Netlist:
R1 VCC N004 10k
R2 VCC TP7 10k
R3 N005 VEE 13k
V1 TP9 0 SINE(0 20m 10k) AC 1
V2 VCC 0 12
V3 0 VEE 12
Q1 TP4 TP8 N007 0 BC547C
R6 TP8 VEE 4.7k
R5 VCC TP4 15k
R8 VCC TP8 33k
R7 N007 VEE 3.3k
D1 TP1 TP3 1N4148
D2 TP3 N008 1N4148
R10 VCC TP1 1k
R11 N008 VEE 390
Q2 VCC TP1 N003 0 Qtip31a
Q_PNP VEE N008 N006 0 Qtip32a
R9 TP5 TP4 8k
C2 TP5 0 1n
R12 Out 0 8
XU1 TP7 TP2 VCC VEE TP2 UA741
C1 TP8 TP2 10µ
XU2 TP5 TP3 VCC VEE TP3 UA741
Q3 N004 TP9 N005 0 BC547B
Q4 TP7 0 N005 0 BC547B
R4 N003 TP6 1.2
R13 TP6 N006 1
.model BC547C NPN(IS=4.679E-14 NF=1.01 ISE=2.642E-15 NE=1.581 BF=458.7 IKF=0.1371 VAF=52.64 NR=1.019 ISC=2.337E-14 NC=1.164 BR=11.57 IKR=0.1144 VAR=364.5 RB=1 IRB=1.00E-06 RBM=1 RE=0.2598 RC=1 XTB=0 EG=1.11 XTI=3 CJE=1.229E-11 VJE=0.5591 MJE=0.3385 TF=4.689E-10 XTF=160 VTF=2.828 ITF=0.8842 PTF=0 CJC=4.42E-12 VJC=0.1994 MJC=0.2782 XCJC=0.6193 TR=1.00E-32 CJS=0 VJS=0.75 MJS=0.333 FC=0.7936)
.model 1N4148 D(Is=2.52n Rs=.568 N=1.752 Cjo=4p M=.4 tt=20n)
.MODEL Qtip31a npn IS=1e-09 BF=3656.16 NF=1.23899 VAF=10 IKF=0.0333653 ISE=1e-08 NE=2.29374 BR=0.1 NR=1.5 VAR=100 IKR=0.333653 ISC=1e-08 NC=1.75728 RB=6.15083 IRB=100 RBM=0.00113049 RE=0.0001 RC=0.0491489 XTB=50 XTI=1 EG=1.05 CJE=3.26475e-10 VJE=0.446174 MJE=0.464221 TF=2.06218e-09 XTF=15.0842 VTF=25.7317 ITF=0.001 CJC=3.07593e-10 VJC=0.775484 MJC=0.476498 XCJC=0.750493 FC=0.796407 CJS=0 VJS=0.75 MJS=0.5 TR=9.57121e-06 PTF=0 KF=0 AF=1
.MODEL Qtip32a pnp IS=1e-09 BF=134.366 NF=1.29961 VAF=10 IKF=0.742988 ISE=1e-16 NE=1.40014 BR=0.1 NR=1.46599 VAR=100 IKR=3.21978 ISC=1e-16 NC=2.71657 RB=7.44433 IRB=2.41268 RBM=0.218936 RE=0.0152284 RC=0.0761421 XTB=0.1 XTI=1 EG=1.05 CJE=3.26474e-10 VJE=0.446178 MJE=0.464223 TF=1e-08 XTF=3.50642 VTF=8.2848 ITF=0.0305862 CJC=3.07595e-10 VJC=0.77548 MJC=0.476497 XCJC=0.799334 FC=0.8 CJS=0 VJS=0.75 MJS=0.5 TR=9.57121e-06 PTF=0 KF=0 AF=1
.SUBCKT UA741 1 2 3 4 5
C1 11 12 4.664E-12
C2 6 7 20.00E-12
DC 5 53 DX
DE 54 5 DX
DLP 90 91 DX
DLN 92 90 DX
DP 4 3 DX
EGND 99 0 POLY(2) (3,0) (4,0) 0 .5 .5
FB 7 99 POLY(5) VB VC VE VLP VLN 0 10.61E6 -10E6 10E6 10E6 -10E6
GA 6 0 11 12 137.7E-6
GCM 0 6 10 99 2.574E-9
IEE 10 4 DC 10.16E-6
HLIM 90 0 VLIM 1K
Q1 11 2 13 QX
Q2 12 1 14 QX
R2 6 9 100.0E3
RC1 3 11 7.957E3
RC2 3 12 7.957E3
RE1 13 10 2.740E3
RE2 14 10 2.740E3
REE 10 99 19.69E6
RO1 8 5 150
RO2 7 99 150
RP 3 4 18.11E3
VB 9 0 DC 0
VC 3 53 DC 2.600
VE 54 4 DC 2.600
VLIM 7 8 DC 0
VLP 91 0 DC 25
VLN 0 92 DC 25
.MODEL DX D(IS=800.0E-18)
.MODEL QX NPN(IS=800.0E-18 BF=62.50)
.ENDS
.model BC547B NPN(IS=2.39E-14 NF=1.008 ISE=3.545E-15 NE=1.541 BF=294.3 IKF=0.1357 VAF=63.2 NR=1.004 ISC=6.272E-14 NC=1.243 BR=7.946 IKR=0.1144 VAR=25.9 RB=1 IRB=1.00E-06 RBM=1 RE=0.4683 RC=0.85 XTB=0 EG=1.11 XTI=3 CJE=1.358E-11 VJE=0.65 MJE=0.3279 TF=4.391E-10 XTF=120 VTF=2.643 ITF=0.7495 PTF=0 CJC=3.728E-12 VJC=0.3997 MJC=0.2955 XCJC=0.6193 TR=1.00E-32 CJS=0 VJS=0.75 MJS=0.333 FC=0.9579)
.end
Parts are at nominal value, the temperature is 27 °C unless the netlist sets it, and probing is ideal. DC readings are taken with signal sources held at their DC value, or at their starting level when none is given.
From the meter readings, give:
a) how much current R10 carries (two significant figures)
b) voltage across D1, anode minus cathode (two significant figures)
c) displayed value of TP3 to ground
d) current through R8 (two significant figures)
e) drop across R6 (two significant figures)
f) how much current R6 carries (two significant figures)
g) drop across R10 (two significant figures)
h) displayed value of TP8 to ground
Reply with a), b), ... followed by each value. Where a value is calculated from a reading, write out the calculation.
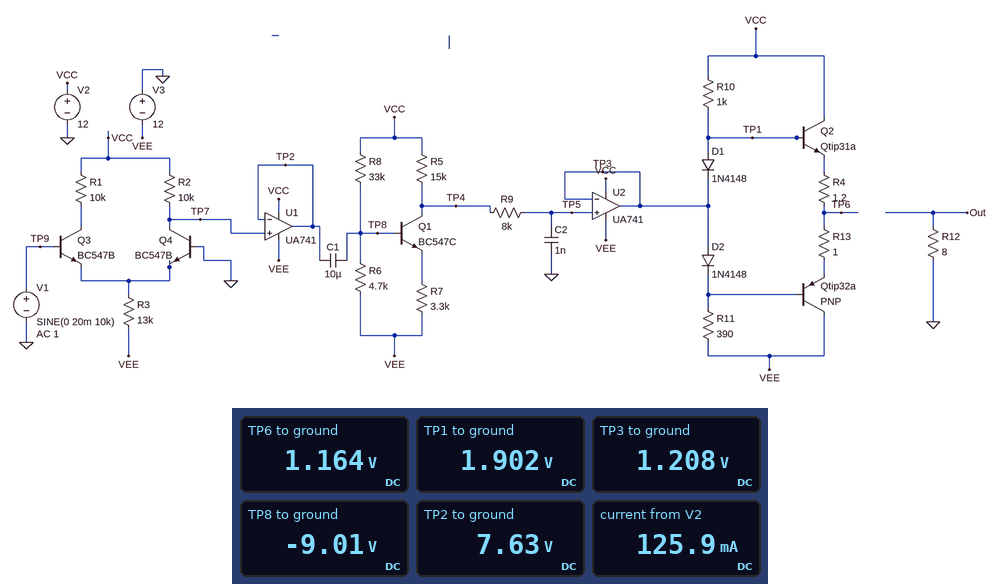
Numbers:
a) (12 V - 1.902 V) / 1 kΩ = 10 mA
b) 1.902 V - 1.208 V = 690 mV
c) 1.208 V
d) (12 V - (-9.01 V)) / 33 kΩ = 640 µA
e) -9.01 V - (-12 V) = 3.0 V
f) (-9.01 V - (-12 V)) / 4.7 kΩ = 640 µA
g) 12 V - 1.902 V = 10 V
h) -9.01 V
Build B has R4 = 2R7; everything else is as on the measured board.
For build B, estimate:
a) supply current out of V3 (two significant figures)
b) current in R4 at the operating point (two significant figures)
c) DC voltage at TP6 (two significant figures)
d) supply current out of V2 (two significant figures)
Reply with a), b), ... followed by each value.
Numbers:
a) 110 mA
b) 76 mA
c) 1.1 V
d) 91 mA
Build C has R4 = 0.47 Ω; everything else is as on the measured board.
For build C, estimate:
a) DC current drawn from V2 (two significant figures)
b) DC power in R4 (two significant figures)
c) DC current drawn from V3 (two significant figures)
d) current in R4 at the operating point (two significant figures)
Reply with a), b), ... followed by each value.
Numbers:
a) 160 mA
b) 10 mW
c) 180 mA
d) 150 mA
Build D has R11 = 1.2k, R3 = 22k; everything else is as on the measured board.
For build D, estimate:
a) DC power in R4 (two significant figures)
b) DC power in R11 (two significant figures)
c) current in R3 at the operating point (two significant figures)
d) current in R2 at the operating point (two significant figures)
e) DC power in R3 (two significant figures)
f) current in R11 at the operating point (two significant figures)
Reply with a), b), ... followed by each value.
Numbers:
a) 9.9 mW
b) 130 mW
c) 520 µA
d) 260 µA
e) 5.9 mW
f) 10 mA
